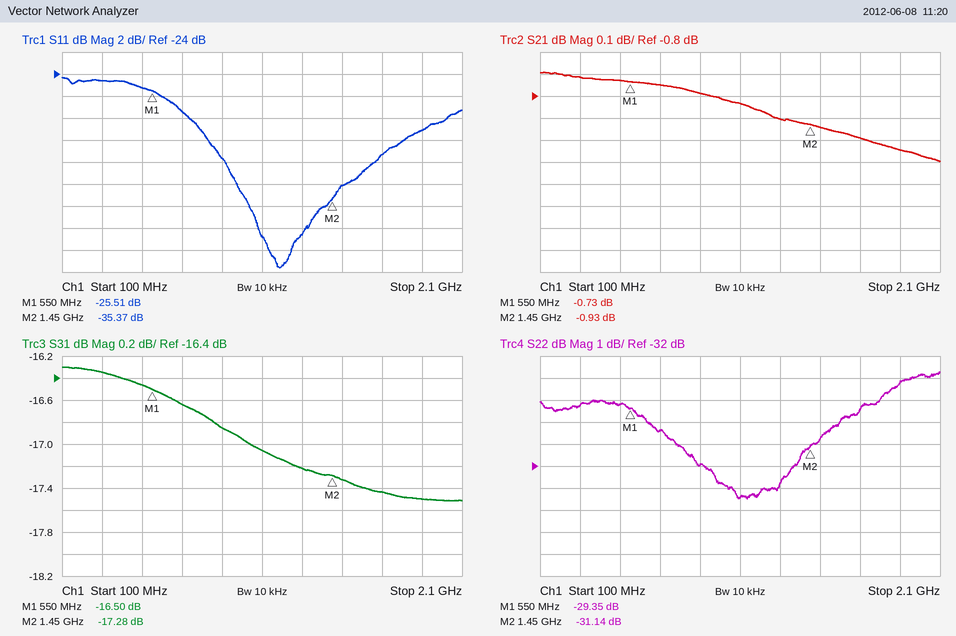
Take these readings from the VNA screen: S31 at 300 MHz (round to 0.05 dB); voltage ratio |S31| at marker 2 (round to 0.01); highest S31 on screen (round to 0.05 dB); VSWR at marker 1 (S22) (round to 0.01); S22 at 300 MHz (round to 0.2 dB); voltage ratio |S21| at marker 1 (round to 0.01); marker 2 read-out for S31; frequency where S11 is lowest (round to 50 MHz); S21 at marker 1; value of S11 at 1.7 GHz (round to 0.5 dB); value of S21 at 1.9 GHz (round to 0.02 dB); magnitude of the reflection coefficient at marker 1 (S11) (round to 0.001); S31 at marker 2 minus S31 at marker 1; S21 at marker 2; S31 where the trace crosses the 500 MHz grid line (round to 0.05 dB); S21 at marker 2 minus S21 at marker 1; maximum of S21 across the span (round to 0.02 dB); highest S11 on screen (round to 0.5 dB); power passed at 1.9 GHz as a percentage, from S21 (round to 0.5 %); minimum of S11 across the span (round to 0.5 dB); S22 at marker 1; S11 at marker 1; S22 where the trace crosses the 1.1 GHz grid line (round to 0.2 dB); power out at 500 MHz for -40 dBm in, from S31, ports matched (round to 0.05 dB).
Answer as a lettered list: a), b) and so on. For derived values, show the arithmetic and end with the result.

a) -16.35 dB
b) 10^(-17.28/20) ≈ 0.14
c) -16.30 dB
d) (1 + 0.0341)/(1 − 0.0341) ≈ 1.07
e) -29.2 dB
f) 10^(-0.73/20) ≈ 0.92
g) -17.28 dB
h) 1.20 GHz
i) -0.73 dB
j) -31.5 dB
k) -1.04 dB
l) 10^(-25.51/20) ≈ 0.053
m) -17.28 − (-16.5) = -0.78 dB
n) -0.93 dB
o) -16.45 dB
p) -0.93 − (-0.73) = -0.20 dB
q) -0.70 dB
r) -24.5 dB
s) 10^(-1.04/10) ≈ 78.7 %, so 78.5 % to the nearest 0.5 %
t) -41.5 dB
u) -29.35 dB
v) -25.51 dB
w) -33.4 dB
x) -40 dBm + (-16.45 dB) = -56.45 dBm
